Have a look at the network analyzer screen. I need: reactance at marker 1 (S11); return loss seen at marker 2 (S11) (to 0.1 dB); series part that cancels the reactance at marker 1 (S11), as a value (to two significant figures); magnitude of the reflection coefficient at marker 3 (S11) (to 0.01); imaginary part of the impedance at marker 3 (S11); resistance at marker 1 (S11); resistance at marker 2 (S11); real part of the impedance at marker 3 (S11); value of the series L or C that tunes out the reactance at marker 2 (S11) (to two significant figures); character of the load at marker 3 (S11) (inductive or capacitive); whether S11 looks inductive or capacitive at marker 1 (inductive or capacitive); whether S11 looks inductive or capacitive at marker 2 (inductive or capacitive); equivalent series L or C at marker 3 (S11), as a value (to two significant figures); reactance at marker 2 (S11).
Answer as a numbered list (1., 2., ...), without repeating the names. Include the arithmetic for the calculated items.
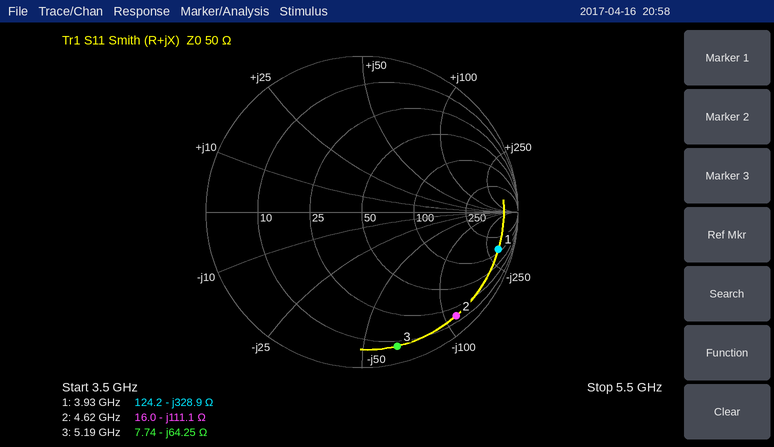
1. -328.9 Ω
2. 0.9 dB
3. L = 328.9 Ω/(2π × 3.93 GHz) ≈ 13 nH
4. 0.89
5. -64.25 Ω
6. 124.2 Ω
7. 16.0 Ω
8. 7.74 Ω
9. L = 111.1 Ω/(2π × 4.62 GHz) ≈ 3.8 nH
10. capacitive
11. capacitive
12. capacitive
13. C = 1/(2π × 5.19 GHz × 64.25 Ω) ≈ 477 fF, so 480 fF to two significant figures
14. -111.1 Ω
